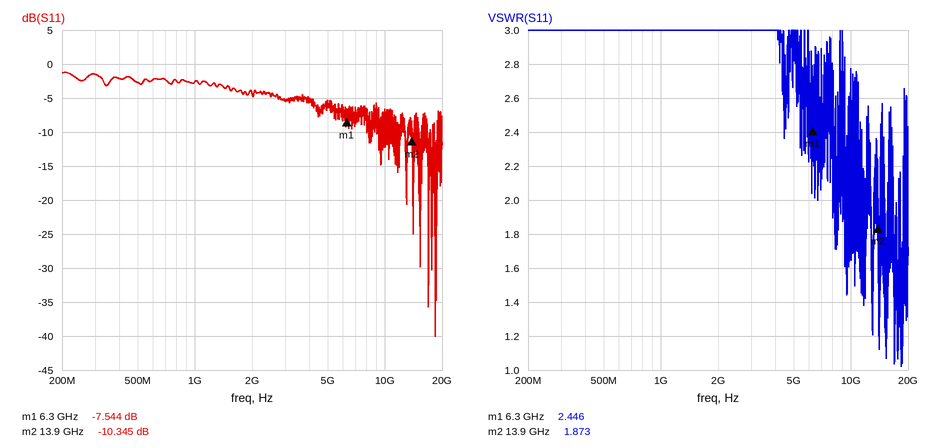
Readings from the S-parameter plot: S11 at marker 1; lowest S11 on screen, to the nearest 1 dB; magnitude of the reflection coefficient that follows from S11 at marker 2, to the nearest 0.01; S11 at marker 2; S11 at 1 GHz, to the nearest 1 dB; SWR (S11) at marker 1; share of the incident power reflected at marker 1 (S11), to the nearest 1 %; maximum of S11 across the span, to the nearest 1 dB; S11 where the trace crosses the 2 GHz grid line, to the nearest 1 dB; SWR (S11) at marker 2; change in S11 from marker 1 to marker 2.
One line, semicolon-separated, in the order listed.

-7.544 dB; -40 dB; 0.30; -10.345 dB; -3 dB; 2.446; 18 %; -1 dB; -4 dB; 1.873; -2.801 dB
